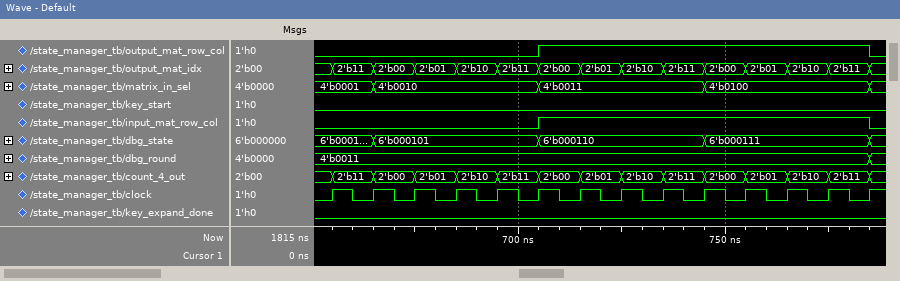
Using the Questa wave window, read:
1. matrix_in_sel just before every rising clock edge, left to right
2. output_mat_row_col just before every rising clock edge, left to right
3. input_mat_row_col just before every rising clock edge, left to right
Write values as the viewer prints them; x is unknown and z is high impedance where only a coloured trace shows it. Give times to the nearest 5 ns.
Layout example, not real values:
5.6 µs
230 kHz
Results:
4'b0001, 4'b0001, 4'b0010, 4'b0010, 4'b0010, 4'b0010, 4'b0011, 4'b0011, 4'b0011, 4'b0011, 4'b0100, 4'b0100, 4'b0100, 4'b0100
0 0 0 0 0 0 1 1 1 1 1 1 1 1
0 0 0 0 0 0 1 1 1 1 1 1 1 1
